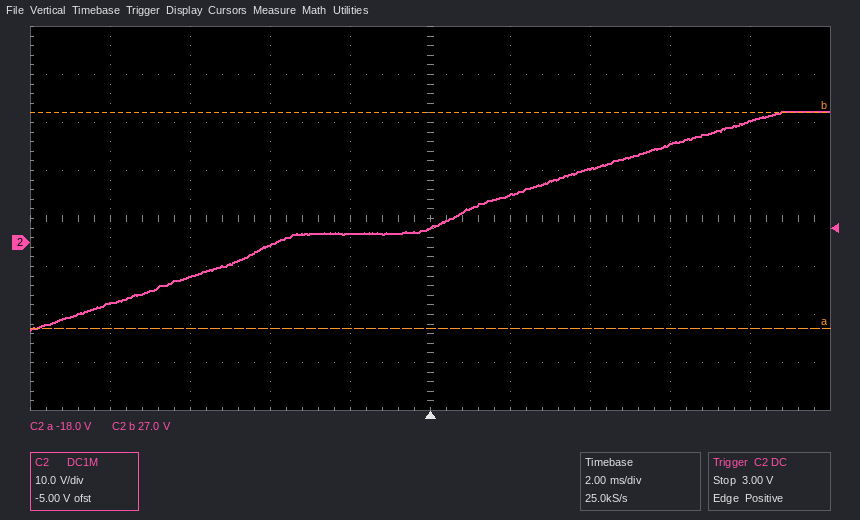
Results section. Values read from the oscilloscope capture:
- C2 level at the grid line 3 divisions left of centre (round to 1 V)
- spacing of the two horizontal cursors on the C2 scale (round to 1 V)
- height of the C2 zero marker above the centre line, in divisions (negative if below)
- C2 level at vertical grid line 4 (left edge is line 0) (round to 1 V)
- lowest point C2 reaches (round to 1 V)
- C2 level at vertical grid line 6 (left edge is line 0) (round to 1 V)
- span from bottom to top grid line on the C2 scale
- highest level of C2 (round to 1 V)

-7 V
45 V
-0.5 div
2 V
-18 V
10 V
80 V
27 V
